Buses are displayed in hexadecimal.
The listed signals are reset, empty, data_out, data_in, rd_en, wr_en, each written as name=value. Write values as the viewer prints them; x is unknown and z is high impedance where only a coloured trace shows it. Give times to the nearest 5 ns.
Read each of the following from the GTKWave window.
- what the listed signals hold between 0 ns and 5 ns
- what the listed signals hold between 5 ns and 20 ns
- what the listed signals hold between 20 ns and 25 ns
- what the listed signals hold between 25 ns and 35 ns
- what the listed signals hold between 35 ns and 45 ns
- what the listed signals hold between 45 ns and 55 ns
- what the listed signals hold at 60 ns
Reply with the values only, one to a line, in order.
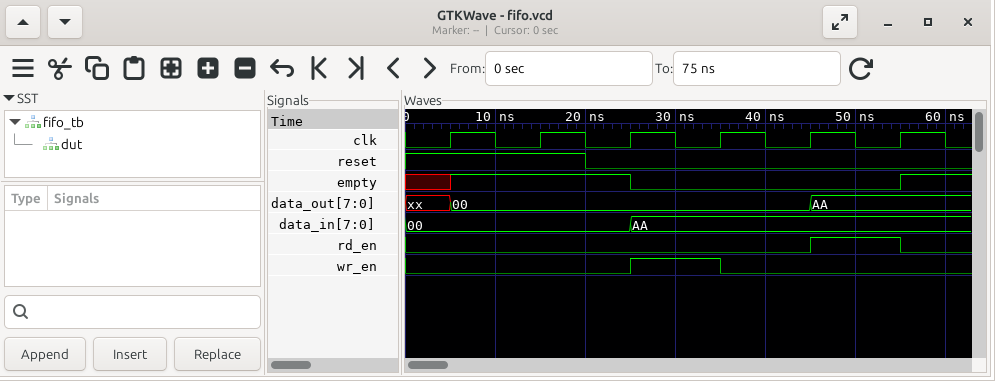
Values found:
reset=1, empty=x, data_out=xx, data_in=00, rd_en=0, wr_en=0
reset=1, empty=1, data_out=00, data_in=00, rd_en=0, wr_en=0
reset=0, empty=1, data_out=00, data_in=00, rd_en=0, wr_en=0
reset=0, empty=0, data_out=00, data_in=AA, rd_en=0, wr_en=1
reset=0, empty=0, data_out=00, data_in=AA, rd_en=0, wr_en=0
reset=0, empty=0, data_out=AA, data_in=AA, rd_en=1, wr_en=0
reset=0, empty=1, data_out=AA, data_in=AA, rd_en=0, wr_en=0
